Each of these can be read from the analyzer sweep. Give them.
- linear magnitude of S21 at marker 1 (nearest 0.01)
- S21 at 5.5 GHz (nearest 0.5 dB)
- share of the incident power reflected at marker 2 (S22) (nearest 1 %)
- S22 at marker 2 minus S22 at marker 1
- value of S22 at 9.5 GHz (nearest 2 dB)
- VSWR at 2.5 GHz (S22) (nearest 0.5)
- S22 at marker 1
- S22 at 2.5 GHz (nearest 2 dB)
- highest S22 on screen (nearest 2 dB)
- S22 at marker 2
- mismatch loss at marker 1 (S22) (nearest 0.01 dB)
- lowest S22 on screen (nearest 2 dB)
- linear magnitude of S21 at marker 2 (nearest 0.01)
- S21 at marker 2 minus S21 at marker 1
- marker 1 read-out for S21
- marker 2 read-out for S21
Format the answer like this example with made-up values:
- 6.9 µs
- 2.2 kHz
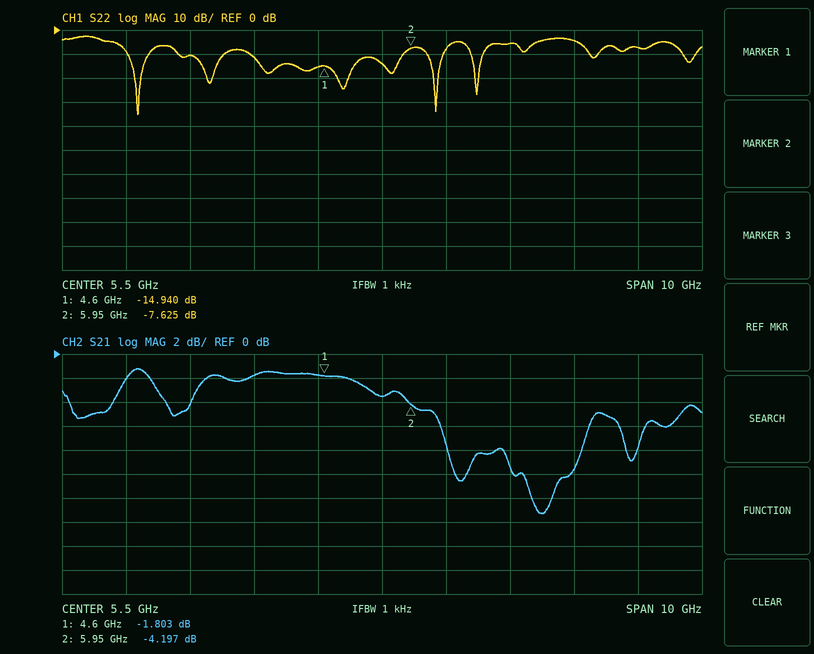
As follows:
- 0.81
- -3.5 dB
- 17 %
- 7.315 dB
- -8 dB
- 2.0
- -14.940 dB
- -10 dB
- -2 dB
- -7.625 dB
- 0.14 dB
- -36 dB
- 0.62
- -2.394 dB
- -1.803 dB
- -4.197 dB
